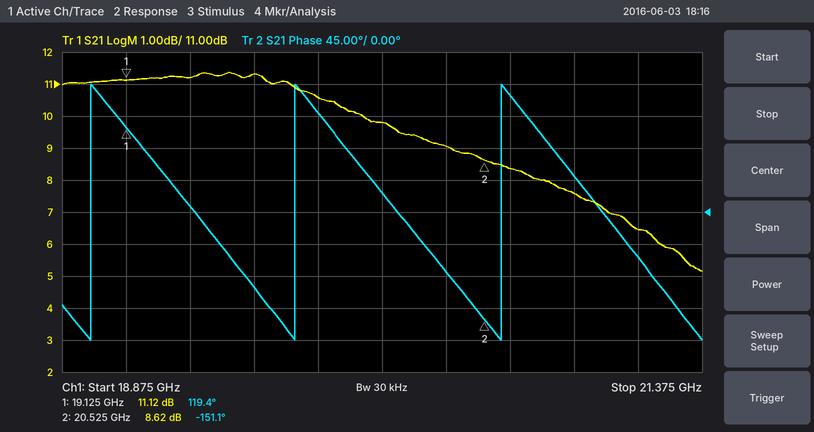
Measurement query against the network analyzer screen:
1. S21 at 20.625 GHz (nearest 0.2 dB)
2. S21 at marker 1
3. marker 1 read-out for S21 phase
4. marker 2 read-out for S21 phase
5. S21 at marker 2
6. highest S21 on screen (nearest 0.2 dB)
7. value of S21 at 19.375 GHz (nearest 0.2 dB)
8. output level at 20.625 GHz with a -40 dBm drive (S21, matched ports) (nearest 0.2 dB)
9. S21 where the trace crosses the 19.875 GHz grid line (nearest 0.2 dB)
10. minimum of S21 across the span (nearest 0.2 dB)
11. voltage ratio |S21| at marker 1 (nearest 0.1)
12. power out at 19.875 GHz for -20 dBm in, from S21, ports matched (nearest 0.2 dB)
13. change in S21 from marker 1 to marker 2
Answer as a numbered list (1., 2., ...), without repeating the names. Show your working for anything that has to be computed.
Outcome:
1. 8.4 dB
2. 11.12 dB
3. 119.4°
4. -151.1°
5. 8.62 dB
6. 11.4 dB
7. 11.2 dB
8. -40 dBm + (8.4 dB) = -31.6 dBm
9. 10.6 dB
10. 5.2 dB
11. 10^(11.12/20) ≈ 3.6
12. -20 dBm + (10.6 dB) = -9.4 dBm
13. 8.62 − (11.12) = -2.50 dB
